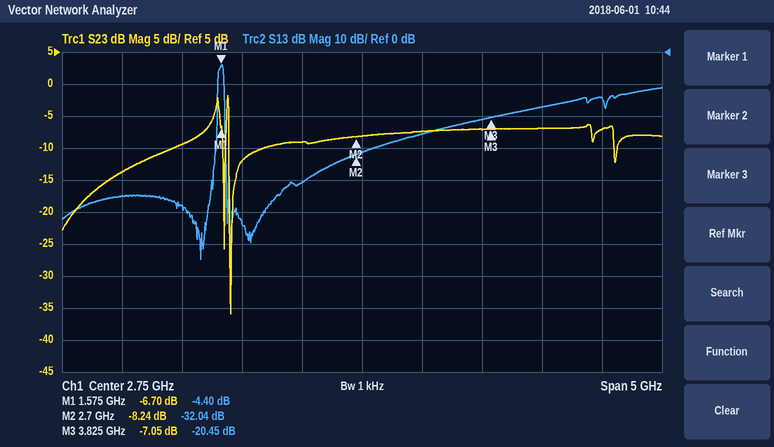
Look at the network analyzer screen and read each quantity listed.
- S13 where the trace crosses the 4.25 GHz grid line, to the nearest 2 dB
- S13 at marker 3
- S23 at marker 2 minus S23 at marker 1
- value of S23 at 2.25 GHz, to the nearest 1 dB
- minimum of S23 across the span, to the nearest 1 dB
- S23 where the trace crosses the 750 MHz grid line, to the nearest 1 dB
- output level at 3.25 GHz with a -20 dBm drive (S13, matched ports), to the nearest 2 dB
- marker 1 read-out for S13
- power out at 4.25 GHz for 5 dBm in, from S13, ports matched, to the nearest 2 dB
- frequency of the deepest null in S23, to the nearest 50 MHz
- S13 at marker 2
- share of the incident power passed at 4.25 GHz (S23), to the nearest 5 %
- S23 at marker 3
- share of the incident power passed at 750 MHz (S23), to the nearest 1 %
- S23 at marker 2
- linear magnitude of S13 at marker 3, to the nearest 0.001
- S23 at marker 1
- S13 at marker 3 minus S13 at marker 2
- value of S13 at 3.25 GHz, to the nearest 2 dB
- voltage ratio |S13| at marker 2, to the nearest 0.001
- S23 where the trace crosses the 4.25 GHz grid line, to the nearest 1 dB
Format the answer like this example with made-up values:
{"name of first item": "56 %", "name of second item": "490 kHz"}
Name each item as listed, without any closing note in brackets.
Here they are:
{"S13 where the trace crosses the 4.25 GHz grid line, to the nearest 2 dB": "-18 dB", "S13 at marker 3": "-20.45 dB", "S23 at marker 2 minus S23 at marker 1": "-1.54 dB", "value of S23 at 2.25 GHz, to the nearest 1 dB": "-9 dB", "minimum of S23 across the span, to the nearest 1 dB": "-36 dB", "S23 where the trace crosses the 750 MHz grid line, to the nearest 1 dB": "-14 dB", "output level at 3.25 GHz with a -20 dBm drive (S13, matched ports), to the nearest 2 dB": "-46 dBm", "marker 1 read-out for S13": "-4.40 dB", "power out at 4.25 GHz for 5 dBm in, from S13, ports matched, to the nearest 2 dB": "-12 dBm", "frequency of the deepest null in S23, to the nearest 50 MHz": "1.65 GHz", "S13 at marker 2": "-32.04 dB", "share of the incident power passed at 4.25 GHz (S23), to the nearest 5 %": "20 %", "S23 at marker 3": "-7.05 dB", "share of the incident power passed at 750 MHz (S23), to the nearest 1 %": "4 %", "S23 at marker 2": "-8.24 dB", "linear magnitude of S13 at marker 3, to the nearest 0.001": "0.095", "S23 at marker 1": "-6.70 dB", "S13 at marker 3 minus S13 at marker 2": "11.59 dB", "value of S13 at 3.25 GHz, to the nearest 2 dB": "-26 dB", "voltage ratio |S13| at marker 2, to the nearest 0.001": "0.025", "S23 where the trace crosses the 4.25 GHz grid line, to the nearest 1 dB": "-7 dB"}
